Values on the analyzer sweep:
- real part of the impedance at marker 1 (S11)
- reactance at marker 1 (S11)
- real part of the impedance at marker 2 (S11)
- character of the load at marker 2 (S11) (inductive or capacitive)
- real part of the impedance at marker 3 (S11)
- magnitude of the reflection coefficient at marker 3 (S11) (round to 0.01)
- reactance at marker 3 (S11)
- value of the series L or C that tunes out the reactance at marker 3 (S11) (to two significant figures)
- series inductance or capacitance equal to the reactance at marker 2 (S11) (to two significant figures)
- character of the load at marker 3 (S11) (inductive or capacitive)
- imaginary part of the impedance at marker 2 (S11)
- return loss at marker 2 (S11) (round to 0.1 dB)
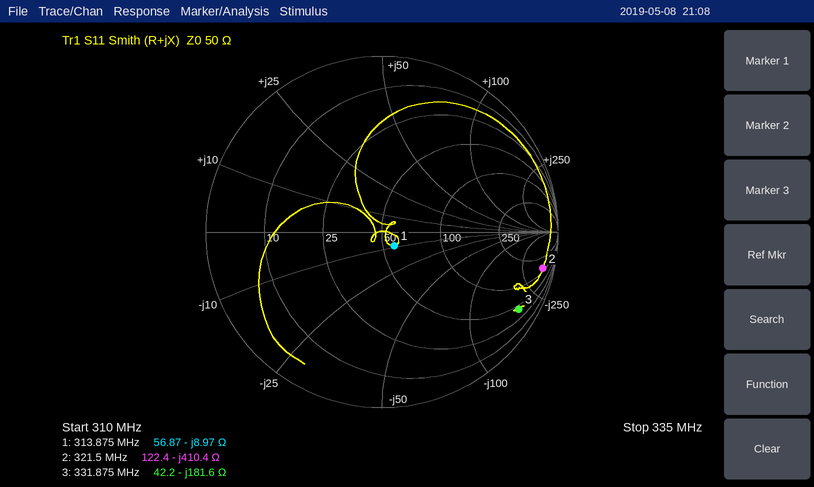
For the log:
56.87 Ω
-8.97 Ω
122.4 Ω
capacitive
42.2 Ω
0.89
-181.6 Ω
87 nH
1.2 pF
capacitive
-410.4 Ω
0.6 dB
